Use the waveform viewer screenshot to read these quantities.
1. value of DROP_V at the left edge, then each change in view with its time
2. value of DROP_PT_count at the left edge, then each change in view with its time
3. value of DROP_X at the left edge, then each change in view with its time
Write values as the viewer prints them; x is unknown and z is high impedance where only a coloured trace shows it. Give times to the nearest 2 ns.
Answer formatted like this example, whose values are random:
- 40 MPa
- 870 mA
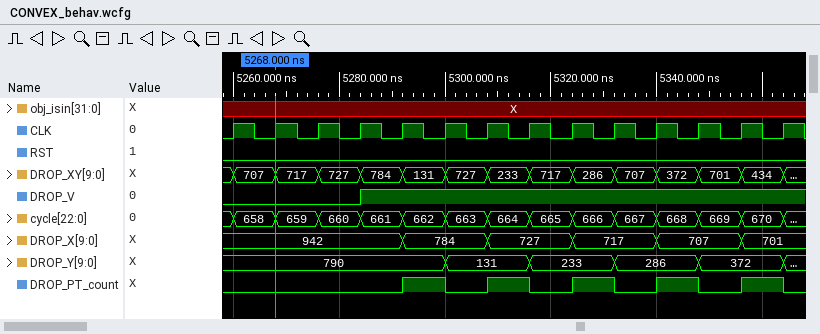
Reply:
- 0, 1 at 5284 ns
- 0, 1 at 5292 ns, 0 at 5300 ns, 1 at 5308 ns, 0 at 5316 ns, 1 at 5324 ns, 0 at 5332 ns, 1 at 5340 ns, 0 at 5348 ns, 1 at 5356 ns, 0 at 5364 ns
- 942, 784 at 5292 ns, 727 at 5308 ns, 717 at 5324 ns, 707 at 5340 ns, 701 at 5356 ns
